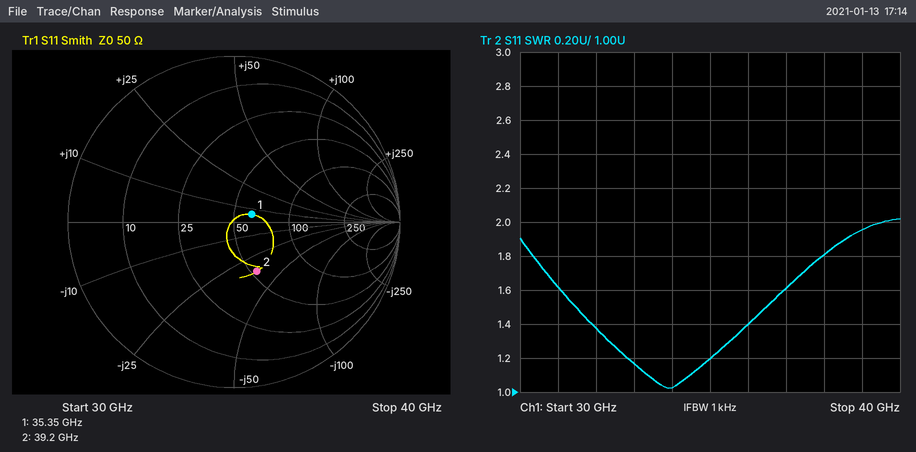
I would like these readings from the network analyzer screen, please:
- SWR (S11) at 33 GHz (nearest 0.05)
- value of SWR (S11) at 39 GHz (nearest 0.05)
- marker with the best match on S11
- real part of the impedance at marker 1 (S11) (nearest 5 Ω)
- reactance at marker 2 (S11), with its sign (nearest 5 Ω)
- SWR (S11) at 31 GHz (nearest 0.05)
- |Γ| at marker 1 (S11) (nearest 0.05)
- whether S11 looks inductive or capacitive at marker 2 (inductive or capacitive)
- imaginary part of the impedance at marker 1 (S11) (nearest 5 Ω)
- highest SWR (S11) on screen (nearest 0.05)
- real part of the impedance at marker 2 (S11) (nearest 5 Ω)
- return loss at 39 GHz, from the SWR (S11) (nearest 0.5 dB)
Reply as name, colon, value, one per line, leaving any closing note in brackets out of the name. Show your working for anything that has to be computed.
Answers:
SWR (S11) at 33 GHz: 1.15
value of SWR (S11) at 39 GHz: 1.95
marker with the best match on S11: marker 1
real part of the impedance at marker 1 (S11): 60 Ω
reactance at marker 2 (S11), with its sign: -35 Ω
SWR (S11) at 31 GHz: 1.60
|Γ| at marker 1 (S11): 0.10
whether S11 looks inductive or capacitive at marker 2: capacitive
imaginary part of the impedance at marker 1 (S11): +5 Ω
highest SWR (S11) on screen: 2.00
real part of the impedance at marker 2 (S11): 55 Ω
return loss at 39 GHz, from the SWR (S11): −20 log10((1.95 − 1)/(1.95 + 1)) ≈ 9.84 dB, so 10.0 dB to the nearest 0.5 dB
